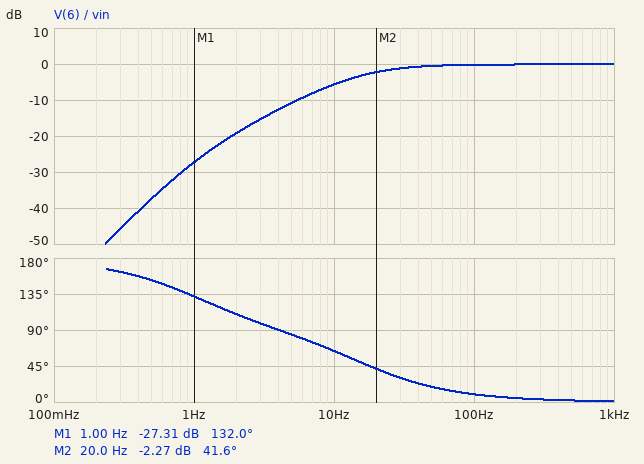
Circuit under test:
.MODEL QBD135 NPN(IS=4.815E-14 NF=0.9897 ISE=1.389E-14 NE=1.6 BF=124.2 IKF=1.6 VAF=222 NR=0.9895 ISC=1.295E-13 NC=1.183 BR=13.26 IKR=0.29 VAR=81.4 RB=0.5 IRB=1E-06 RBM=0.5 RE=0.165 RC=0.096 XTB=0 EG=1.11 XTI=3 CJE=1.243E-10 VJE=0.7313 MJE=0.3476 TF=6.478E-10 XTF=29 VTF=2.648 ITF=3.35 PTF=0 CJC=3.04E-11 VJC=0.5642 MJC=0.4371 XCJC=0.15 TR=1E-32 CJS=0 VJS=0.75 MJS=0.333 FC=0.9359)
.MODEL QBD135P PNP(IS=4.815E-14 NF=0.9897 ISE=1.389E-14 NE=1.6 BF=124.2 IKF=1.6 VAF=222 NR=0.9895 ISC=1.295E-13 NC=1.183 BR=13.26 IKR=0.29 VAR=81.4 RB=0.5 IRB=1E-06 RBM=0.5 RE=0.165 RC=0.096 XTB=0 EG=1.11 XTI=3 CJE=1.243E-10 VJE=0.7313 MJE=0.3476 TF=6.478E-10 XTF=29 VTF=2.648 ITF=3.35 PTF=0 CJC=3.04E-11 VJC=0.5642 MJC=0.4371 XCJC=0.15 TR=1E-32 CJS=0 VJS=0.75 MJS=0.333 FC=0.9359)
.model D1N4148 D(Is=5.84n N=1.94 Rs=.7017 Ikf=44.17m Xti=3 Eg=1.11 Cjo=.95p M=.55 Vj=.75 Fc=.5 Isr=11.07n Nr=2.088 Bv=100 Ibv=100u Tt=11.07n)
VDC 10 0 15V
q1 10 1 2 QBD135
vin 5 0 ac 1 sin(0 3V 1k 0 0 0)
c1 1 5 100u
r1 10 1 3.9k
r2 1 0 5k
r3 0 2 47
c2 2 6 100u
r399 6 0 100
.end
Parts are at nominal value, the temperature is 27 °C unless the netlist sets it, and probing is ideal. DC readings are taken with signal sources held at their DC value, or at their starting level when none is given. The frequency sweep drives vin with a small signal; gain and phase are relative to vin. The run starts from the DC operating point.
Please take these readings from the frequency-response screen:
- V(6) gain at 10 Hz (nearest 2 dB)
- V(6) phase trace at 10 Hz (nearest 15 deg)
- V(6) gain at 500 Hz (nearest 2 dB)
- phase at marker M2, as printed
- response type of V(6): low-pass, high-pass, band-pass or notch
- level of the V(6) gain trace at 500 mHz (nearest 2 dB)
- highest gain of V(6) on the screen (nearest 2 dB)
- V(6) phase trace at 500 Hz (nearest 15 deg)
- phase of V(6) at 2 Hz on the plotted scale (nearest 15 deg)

-6 dB
60 deg
0 dB
41.6 deg
high-pass
-38 dB
0 dB
0 deg
105 deg
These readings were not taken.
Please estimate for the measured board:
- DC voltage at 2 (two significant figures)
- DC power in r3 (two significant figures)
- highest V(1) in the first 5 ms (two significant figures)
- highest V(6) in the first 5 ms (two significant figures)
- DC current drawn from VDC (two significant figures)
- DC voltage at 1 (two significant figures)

5.5 V
650 mW
9.3 V
2.9 V
120 mA
6.3 V
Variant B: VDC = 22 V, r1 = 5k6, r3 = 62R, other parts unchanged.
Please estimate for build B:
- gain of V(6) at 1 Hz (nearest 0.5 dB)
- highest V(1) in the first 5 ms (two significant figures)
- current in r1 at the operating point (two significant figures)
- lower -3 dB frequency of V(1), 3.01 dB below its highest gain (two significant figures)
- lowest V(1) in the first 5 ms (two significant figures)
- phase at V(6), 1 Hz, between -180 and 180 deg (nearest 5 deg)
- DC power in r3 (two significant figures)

-26.5 dB
11 V
2.5 mA
840 mHz
4.9 V
125 deg
830 mW
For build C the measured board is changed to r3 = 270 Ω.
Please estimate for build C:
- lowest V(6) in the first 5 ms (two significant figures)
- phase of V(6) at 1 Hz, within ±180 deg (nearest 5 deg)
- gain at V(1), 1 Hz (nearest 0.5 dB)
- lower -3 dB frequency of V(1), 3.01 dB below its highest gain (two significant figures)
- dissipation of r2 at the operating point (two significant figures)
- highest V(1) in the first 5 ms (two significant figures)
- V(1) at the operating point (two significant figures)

-2.0 V
125 deg
-2.0 dB
780 mHz
13 mW
11 V
8.0 V
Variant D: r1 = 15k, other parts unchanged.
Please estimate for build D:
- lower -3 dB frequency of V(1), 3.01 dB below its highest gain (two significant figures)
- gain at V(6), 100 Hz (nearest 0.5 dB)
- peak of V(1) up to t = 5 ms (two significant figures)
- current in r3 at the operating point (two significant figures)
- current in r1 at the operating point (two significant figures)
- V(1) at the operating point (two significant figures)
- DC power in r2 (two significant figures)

700 mHz
-0.5 dB
5.6 V
40 mA
830 µA
2.6 V
1.3 mW
